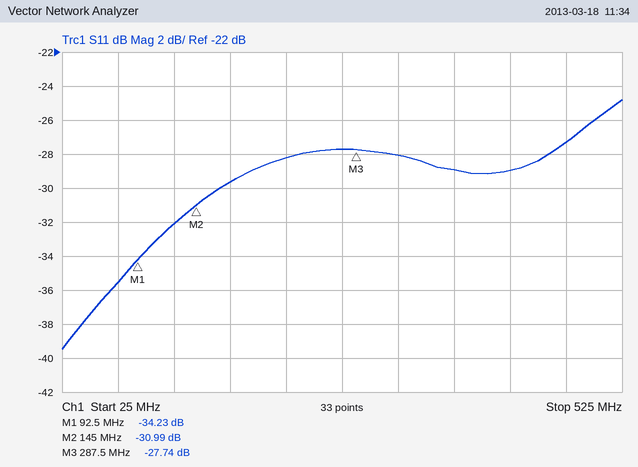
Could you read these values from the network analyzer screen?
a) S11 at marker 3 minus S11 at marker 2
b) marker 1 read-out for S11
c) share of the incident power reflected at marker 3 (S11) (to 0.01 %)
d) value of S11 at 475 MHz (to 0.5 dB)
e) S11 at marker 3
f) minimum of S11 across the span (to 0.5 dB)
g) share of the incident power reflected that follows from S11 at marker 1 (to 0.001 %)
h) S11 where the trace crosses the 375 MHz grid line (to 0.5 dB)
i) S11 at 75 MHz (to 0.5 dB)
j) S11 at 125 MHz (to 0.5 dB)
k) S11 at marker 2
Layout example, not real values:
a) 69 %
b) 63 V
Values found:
a) 3.25 dB
b) -34.23 dB
c) 0.17 %
d) -27.5 dB
e) -27.74 dB
f) -39.5 dB
g) 0.038 %
h) -29.0 dB
i) -35.5 dB
j) -32.0 dB
k) -30.99 dB
